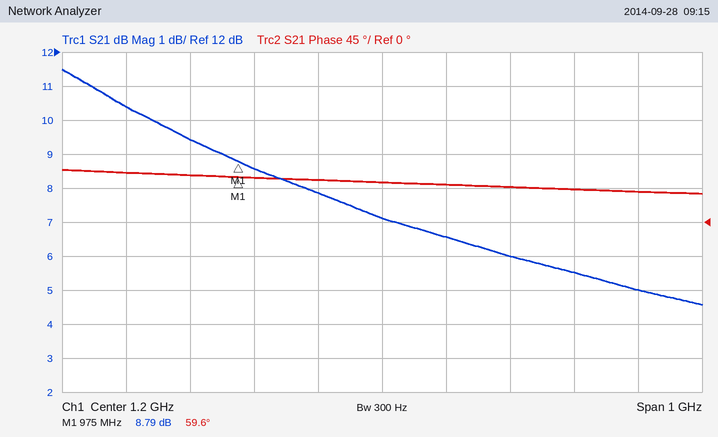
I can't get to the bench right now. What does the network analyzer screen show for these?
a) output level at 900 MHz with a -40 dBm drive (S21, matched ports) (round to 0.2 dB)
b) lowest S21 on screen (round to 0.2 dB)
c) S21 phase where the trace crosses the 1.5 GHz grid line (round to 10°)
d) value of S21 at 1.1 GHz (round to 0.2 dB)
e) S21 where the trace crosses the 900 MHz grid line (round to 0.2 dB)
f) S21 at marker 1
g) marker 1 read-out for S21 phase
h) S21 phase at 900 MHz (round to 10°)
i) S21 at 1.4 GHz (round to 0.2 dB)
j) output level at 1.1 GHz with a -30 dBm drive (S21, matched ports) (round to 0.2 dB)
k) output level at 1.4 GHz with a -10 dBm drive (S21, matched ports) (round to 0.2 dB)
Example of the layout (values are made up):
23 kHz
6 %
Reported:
-30.6 dBm
4.6 dB
40°
7.8 dB
9.4 dB
8.79 dB
59.6°
60°
6.0 dB
-22.2 dBm
-4.0 dBm
